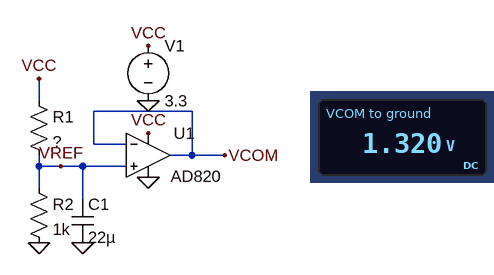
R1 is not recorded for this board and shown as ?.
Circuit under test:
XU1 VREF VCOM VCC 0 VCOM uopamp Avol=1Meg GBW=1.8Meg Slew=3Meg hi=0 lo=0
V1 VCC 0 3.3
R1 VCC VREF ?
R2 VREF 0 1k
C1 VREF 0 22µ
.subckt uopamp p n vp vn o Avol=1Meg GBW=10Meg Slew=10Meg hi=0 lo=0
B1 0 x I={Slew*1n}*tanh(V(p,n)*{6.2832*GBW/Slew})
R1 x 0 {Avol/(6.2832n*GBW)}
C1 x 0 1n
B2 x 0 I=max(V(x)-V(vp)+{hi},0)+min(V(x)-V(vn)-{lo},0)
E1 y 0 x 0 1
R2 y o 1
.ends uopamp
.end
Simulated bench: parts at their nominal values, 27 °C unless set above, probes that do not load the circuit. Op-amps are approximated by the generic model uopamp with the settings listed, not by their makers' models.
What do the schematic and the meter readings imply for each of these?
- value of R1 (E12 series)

1.5 kΩ
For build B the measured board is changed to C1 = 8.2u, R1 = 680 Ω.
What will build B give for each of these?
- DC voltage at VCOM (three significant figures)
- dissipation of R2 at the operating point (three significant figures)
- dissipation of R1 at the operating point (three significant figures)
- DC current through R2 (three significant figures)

1.96 V
3.86 mW
2.62 mW
1.96 mA
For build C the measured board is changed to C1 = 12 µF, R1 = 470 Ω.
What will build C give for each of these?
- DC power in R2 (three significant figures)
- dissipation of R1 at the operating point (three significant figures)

5.04 mW
2.37 mW
